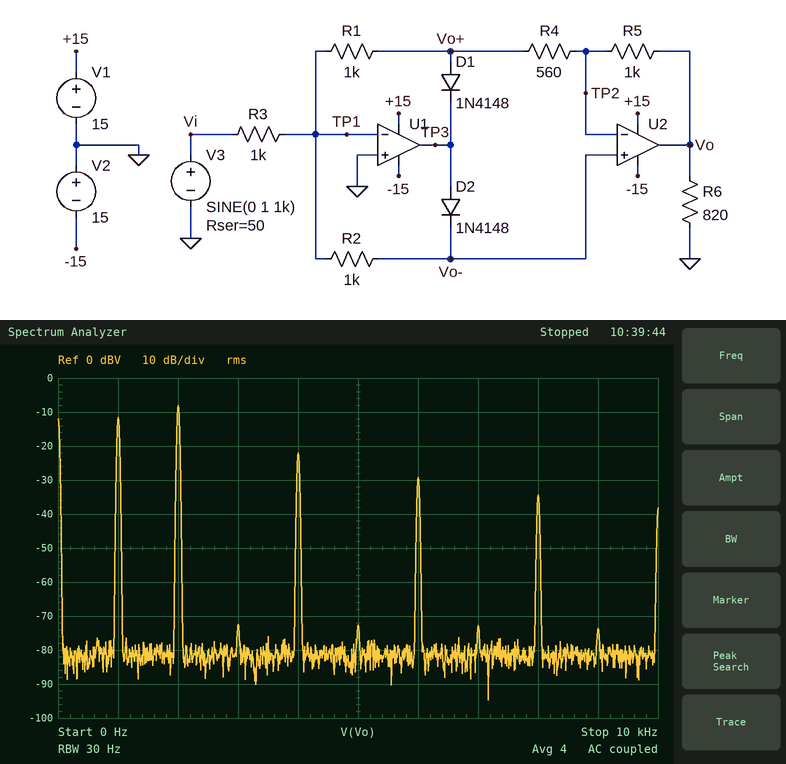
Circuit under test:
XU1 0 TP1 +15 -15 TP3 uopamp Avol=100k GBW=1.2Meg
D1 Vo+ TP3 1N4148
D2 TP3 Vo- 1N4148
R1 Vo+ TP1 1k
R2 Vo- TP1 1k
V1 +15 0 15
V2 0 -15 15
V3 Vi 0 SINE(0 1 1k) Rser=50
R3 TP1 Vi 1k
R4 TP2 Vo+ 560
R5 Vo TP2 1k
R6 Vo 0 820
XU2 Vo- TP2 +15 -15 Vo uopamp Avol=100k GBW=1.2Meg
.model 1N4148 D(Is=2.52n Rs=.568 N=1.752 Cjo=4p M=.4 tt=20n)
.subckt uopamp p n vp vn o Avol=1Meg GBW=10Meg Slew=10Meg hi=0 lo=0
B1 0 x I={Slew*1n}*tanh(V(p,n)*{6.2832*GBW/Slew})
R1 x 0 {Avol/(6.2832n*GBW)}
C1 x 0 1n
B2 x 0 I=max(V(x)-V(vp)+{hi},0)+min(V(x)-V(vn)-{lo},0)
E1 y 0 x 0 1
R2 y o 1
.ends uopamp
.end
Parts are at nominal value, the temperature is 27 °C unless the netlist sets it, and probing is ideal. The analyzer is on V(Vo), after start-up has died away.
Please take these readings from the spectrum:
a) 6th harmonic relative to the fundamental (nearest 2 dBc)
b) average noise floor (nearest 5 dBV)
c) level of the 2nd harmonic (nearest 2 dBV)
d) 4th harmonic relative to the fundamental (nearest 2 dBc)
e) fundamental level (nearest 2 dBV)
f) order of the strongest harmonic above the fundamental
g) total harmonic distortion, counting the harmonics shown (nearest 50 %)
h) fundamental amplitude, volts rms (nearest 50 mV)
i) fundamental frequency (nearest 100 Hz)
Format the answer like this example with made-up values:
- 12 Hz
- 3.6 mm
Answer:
- -18 dBc
- -80 dBV
- -8 dBV
- -10 dBc
- -12 dBV
- 2
- 150 %
- 250 mV
- 1.0 kHz
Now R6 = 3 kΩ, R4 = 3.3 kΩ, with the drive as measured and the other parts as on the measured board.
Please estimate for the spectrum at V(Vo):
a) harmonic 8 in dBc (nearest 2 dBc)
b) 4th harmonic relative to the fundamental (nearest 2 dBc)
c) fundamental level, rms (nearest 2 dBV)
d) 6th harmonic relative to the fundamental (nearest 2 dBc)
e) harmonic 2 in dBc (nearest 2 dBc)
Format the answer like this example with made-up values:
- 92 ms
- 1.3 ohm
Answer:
- -28 dBc
- -16 dBc
- -12 dBV
- -24 dBc
- -2 dBc
